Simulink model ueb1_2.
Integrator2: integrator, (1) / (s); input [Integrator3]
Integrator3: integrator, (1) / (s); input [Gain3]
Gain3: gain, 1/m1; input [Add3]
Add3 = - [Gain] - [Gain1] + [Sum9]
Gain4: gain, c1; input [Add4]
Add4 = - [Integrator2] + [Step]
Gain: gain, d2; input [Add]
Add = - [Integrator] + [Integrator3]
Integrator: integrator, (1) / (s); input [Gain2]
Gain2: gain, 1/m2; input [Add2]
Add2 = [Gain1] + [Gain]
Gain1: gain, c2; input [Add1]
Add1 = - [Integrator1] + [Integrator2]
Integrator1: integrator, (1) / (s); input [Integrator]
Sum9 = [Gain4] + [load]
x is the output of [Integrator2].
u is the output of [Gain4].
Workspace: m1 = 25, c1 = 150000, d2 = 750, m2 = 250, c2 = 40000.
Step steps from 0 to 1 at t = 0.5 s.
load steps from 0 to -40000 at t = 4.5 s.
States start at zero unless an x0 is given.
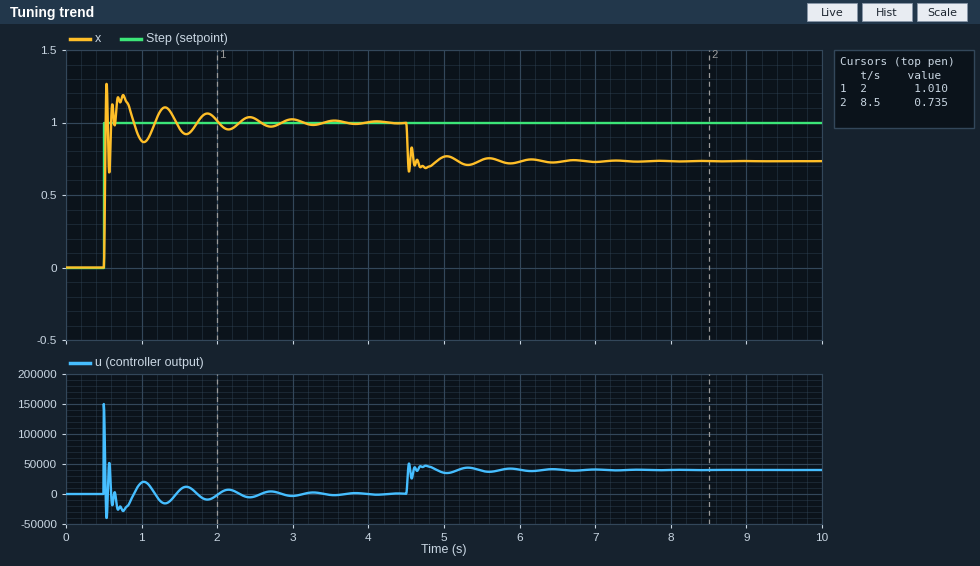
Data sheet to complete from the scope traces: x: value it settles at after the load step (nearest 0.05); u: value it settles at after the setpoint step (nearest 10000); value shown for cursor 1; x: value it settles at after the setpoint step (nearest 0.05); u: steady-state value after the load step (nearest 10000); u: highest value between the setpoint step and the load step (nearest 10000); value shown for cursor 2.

0.75
0
1.010
1.00
40000
150000
0.735
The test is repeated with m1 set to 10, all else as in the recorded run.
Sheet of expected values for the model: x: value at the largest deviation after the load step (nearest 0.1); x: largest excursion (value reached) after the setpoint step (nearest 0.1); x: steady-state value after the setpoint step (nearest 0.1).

0.7
1.2
1.0
